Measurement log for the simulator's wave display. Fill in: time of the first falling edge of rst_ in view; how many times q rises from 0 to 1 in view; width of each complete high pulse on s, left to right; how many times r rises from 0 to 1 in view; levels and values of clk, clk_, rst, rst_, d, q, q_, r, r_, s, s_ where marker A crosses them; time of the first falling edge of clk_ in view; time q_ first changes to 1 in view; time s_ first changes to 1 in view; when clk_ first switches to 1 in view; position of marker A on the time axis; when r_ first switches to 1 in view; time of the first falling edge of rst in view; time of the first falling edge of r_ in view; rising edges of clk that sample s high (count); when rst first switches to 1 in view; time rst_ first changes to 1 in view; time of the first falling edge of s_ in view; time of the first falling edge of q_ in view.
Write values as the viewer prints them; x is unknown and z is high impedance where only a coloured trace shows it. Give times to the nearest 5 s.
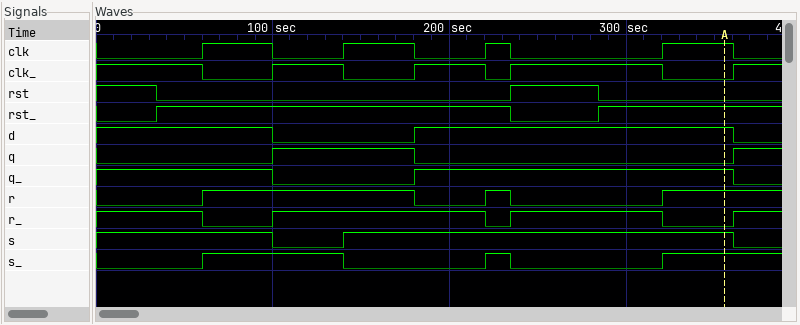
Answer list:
235 s
2
220 s
3
clk=1, clk_=0, rst=0, rst_=1, d=1, q=0, q_=1, r=1, r_=0, s=1, s_=1
60 s
180 s
60 s
100 s
355 s
100 s
35 s
60 s
3
235 s
35 s
140 s
100 s
